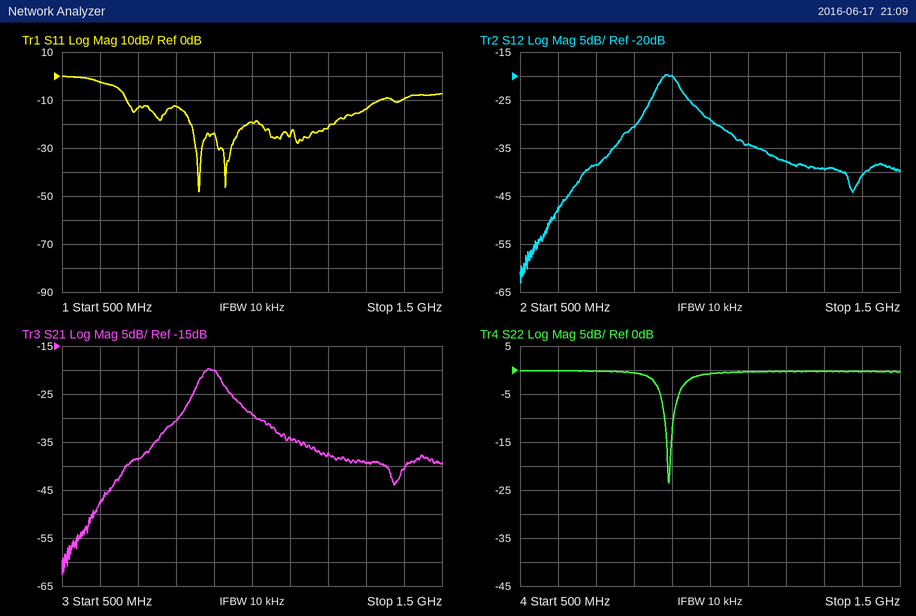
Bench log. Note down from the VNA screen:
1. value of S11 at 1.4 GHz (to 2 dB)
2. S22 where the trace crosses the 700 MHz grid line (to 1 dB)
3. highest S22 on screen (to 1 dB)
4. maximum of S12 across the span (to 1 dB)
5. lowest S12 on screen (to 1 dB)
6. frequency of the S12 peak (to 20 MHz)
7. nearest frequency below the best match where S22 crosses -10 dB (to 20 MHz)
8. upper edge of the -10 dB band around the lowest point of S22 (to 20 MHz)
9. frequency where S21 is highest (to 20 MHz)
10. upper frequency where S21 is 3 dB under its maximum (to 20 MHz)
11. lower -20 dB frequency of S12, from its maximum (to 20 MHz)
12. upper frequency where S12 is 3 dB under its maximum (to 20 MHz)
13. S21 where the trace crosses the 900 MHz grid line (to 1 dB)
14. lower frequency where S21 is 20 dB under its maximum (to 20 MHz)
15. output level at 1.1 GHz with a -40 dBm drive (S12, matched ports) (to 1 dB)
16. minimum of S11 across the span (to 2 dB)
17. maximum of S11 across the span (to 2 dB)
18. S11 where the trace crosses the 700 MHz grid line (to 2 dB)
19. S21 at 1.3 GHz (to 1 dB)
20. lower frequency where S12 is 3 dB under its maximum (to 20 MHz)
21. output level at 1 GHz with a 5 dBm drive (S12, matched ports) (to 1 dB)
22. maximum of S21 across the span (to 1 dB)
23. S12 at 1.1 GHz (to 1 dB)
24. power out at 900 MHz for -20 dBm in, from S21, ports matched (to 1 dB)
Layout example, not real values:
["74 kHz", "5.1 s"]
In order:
["-10 dB", "0 dB", "0 dB", "-20 dB", "-63 dB", "880 MHz", "880 MHz", "900 MHz", "880 MHz", "920 MHz", "680 MHz", "920 MHz", "-20 dB", "680 MHz", "-74 dBm", "-48 dB", "0 dB", "-14 dB", "-39 dB", "860 MHz", "-24 dBm", "-20 dB", "-34 dB", "-40 dBm"]
